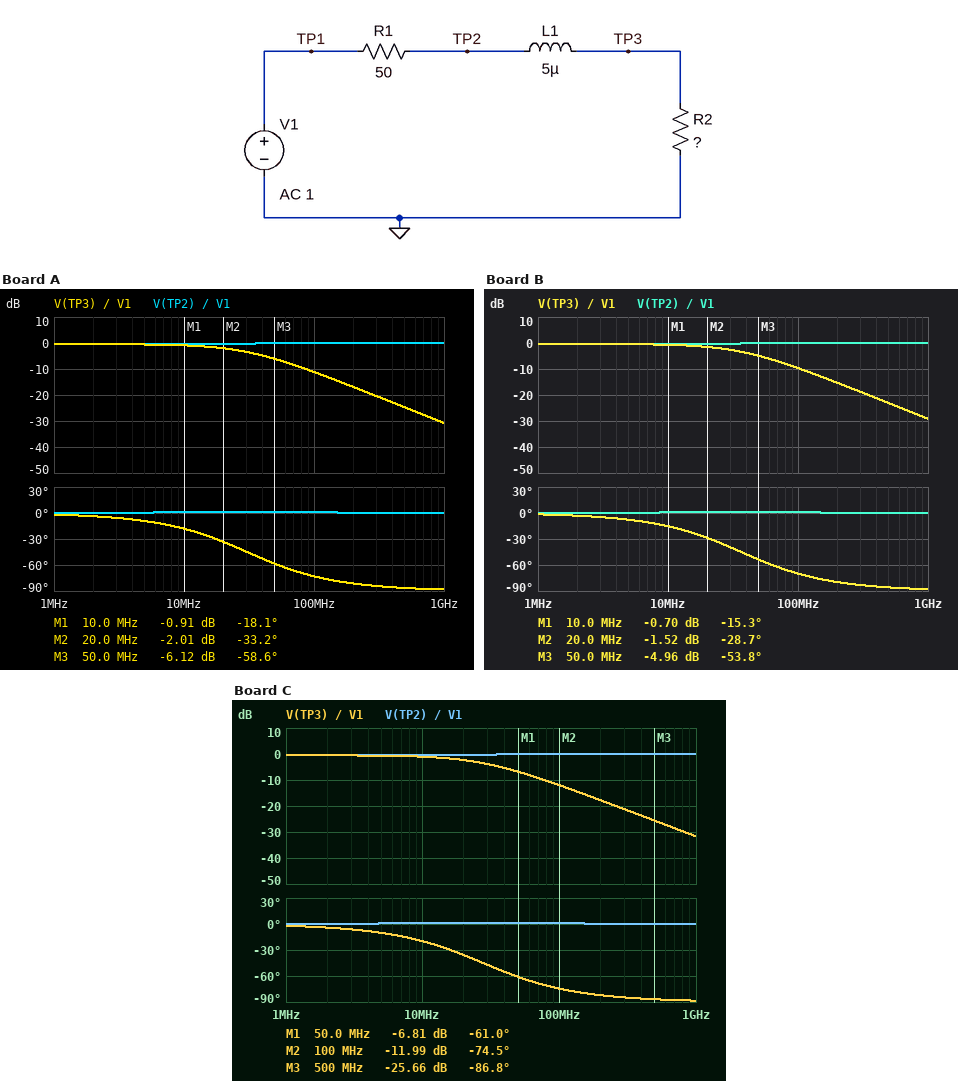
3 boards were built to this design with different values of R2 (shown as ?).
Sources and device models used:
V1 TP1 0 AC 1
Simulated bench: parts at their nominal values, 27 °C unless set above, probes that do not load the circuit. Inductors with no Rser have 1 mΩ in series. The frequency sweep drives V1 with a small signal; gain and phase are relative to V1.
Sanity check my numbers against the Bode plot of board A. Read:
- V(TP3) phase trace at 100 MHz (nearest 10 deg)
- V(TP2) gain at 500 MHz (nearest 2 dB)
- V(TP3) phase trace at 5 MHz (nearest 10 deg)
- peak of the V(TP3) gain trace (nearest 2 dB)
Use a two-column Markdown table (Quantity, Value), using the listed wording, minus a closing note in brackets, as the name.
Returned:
| Quantity | Value |
|---|---|
| V(TP3) phase trace at 100 MHz | -70 deg |
| V(TP2) gain at 500 MHz | 0 dB |
| V(TP3) phase trace at 5 MHz | -10 deg |
| peak of the V(TP3) gain trace | 0 dB |
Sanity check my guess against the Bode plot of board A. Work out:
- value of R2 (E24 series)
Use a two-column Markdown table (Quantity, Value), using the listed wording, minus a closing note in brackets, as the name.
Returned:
| Quantity | Value |
|---|---|
| value of R2 | 910 Ω |
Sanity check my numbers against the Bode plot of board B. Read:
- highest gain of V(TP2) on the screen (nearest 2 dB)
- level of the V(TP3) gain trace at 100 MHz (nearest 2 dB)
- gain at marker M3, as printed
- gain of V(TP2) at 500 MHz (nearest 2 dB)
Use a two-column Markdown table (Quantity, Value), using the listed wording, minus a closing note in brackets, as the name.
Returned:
| Quantity | Value |
|---|---|
| highest gain of V(TP2) on the screen | 0 dB |
| level of the V(TP3) gain trace at 100 MHz | -10 dB |
| gain at marker M3, as printed | -4.96 dB |
| gain of V(TP2) at 500 MHz | 0 dB |
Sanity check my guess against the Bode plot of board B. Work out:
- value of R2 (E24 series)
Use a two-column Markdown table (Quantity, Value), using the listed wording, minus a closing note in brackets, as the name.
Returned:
| Quantity | Value |
|---|---|
| value of R2 | 1.1 kΩ |
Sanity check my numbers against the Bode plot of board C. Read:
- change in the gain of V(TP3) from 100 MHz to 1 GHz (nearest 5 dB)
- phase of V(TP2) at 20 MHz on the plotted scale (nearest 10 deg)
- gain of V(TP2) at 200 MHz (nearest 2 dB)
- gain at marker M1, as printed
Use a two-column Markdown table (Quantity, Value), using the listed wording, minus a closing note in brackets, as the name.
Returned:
| Quantity | Value |
|---|---|
| change in the gain of V(TP3) from 100 MHz to 1 GHz | -20 dB |
| phase of V(TP2) at 20 MHz on the plotted scale | 0 deg |
| gain of V(TP2) at 200 MHz | 0 dB |
| gain at marker M1, as printed | -6.81 dB |
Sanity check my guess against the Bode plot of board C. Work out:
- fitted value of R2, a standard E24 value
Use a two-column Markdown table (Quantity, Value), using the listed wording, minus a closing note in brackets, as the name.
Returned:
| Quantity | Value |
|---|---|
| fitted value of R2, a standard E24 value | 820 Ω |
